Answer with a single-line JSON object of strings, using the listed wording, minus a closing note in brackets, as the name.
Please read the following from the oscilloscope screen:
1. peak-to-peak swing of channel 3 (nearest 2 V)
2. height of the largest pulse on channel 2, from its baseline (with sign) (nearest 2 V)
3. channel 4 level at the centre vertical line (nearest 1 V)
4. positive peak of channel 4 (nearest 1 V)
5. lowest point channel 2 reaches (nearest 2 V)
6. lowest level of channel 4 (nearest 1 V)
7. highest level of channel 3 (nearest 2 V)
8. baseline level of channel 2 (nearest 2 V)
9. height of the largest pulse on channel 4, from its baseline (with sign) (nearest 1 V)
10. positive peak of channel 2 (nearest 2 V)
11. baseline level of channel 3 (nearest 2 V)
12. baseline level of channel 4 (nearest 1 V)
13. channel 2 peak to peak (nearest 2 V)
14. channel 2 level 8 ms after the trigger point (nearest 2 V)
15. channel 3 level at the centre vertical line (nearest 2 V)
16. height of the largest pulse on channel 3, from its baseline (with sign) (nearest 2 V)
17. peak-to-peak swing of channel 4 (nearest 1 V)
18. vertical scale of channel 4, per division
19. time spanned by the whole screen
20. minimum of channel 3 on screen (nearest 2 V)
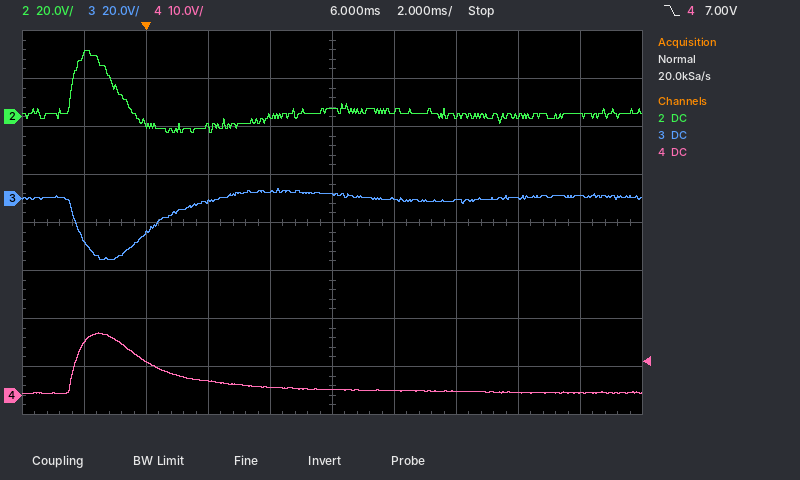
{"peak-to-peak swing of channel 3": "30 V", "height of the largest pulse on channel 2, from its baseline (with sign)": "+26 V", "channel 4 level at the centre vertical line": "1 V", "positive peak of channel 4": "13 V", "lowest point channel 2 reaches": "-6 V", "lowest level of channel 4": "0 V", "highest level of channel 3": "4 V", "baseline level of channel 2": "2 V", "height of the largest pulse on channel 4, from its baseline (with sign)": "+12 V", "positive peak of channel 2": "28 V", "baseline level of channel 3": "0 V", "baseline level of channel 4": "1 V", "channel 2 peak to peak": "34 V", "channel 2 level 8 ms after the trigger point": "2 V", "channel 3 level at the centre vertical line": "2 V", "height of the largest pulse on channel 3, from its baseline (with sign)": "-26 V", "peak-to-peak swing of channel 4": "13 V", "vertical scale of channel 4, per division": "10 V", "time spanned by the whole screen": "20 ms", "minimum of channel 3 on screen": "-26 V"}
